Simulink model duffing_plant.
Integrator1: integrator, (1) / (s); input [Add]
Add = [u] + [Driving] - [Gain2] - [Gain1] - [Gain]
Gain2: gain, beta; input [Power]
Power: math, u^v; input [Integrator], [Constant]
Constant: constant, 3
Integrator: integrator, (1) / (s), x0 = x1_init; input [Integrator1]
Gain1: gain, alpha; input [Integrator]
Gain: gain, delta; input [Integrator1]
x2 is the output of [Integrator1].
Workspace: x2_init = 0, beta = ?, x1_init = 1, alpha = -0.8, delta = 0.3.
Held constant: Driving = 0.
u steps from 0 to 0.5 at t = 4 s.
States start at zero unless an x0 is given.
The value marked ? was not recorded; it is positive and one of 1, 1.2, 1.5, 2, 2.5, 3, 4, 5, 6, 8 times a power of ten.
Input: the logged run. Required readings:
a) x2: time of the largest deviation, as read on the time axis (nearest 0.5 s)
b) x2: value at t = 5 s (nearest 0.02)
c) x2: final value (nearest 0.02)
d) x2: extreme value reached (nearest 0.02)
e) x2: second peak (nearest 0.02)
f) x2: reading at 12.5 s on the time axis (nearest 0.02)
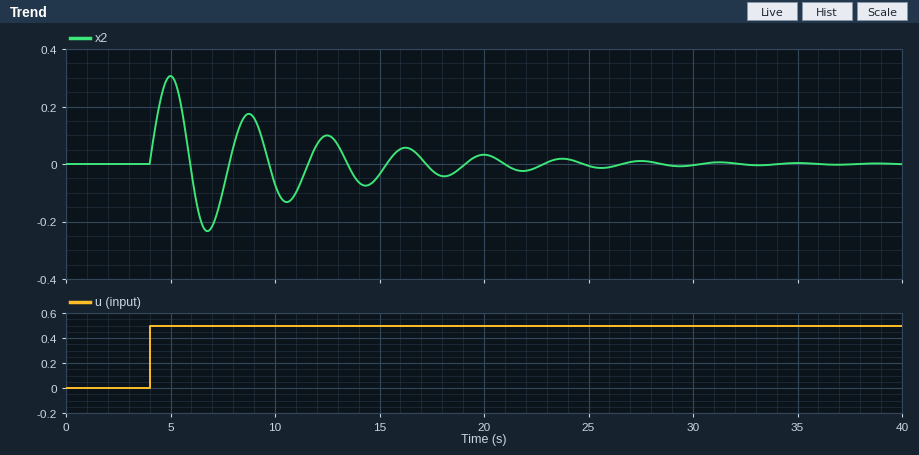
5.0 s
0.30
0.00
0.30
0.18
0.10
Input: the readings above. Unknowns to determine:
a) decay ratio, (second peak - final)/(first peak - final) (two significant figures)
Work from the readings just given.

0.60
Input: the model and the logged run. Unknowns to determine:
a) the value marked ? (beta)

0.8
